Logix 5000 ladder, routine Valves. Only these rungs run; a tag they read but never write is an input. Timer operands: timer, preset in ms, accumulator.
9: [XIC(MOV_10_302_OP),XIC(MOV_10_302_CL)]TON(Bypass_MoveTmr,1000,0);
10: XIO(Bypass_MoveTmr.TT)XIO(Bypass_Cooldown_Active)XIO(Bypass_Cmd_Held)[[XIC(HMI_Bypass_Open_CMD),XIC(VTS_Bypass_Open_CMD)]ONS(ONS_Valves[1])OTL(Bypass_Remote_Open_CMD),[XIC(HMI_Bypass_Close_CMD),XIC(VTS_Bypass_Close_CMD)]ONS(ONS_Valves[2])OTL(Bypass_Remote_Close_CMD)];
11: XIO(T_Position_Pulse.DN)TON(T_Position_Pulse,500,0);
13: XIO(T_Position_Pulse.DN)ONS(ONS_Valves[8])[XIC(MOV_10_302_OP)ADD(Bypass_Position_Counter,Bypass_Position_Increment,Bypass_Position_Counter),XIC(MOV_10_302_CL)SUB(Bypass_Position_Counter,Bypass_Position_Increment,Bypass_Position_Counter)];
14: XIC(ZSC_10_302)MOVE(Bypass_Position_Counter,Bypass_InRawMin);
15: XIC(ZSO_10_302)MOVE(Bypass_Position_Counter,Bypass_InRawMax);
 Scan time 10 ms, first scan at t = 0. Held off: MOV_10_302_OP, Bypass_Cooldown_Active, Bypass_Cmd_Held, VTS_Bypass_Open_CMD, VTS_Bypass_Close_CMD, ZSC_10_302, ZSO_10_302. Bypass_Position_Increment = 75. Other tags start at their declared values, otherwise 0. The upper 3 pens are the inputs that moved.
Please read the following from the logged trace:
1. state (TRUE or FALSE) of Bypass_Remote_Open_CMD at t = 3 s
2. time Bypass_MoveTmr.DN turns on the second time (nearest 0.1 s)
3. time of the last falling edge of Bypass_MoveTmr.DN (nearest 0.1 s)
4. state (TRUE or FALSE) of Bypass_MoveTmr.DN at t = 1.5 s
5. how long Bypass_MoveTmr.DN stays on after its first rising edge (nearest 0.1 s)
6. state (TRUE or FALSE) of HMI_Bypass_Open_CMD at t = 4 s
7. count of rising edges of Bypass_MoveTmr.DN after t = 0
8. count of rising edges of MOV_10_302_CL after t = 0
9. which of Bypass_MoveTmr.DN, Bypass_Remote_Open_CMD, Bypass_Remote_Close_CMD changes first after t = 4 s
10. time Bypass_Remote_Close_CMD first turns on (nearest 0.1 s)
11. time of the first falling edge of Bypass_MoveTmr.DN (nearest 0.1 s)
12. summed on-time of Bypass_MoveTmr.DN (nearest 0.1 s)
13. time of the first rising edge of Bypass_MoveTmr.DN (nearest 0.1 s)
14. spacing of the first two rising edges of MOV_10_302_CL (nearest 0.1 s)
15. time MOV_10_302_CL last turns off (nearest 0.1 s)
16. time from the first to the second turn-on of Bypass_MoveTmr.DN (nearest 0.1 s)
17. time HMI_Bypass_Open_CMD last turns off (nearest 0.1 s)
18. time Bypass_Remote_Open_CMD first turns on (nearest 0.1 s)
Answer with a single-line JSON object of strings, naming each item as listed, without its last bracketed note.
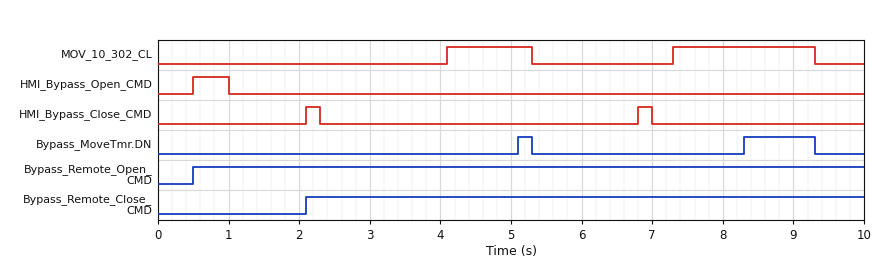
{"state (TRUE or FALSE) of Bypass_Remote_Open_CMD at t = 3 s": "TRUE", "time Bypass_MoveTmr.DN turns on the second time": "8.3 s", "time of the last falling edge of Bypass_MoveTmr.DN": "9.3 s", "state (TRUE or FALSE) of Bypass_MoveTmr.DN at t = 1.5 s": "FALSE", "how long Bypass_MoveTmr.DN stays on after its first rising edge": "0.2 s", "state (TRUE or FALSE) of HMI_Bypass_Open_CMD at t = 4 s": "FALSE", "count of rising edges of Bypass_MoveTmr.DN after t = 0": "2", "count of rising edges of MOV_10_302_CL after t = 0": "2", "which of Bypass_MoveTmr.DN, Bypass_Remote_Open_CMD, Bypass_Remote_Close_CMD changes first after t = 4 s": "Bypass_MoveTmr.DN", "time Bypass_Remote_Close_CMD first turns on": "2.1 s", "time of the first falling edge of Bypass_MoveTmr.DN": "5.3 s", "summed on-time of Bypass_MoveTmr.DN": "1.2 s", "time of the first rising edge of Bypass_MoveTmr.DN": "5.1 s", "spacing of the first two rising edges of MOV_10_302_CL": "3.2 s", "time MOV_10_302_CL last turns off": "9.3 s", "time from the first to the second turn-on of Bypass_MoveTmr.DN": "3.2 s", "time HMI_Bypass_Open_CMD last turns off": "1.0 s", "time Bypass_Remote_Open_CMD first turns on": "0.5 s"}
